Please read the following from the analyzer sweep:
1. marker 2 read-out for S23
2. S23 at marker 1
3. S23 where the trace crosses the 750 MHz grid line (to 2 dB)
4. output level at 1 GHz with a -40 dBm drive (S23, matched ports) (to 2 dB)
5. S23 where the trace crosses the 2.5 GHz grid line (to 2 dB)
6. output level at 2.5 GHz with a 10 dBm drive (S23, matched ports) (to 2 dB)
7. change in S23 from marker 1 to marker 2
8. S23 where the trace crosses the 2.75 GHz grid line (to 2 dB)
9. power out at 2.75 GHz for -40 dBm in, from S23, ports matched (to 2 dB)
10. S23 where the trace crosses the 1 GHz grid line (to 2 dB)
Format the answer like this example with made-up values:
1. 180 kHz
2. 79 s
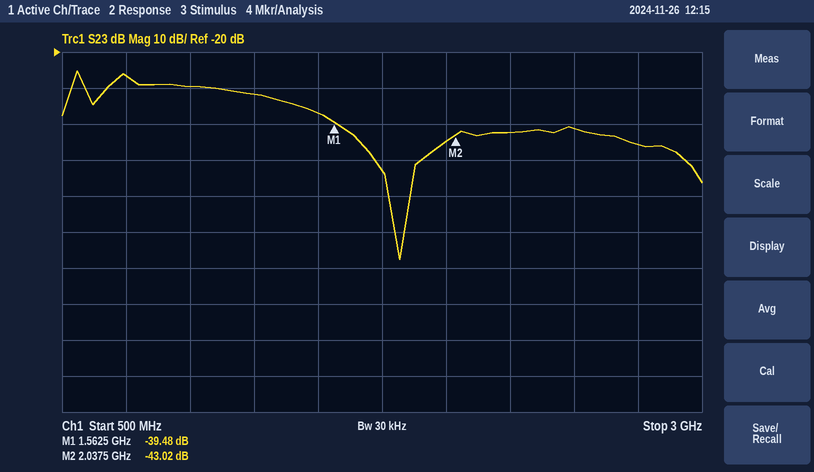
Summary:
1. -43.02 dB
2. -39.48 dB
3. -26 dB
4. -70 dBm
5. -42 dB
6. -32 dBm
7. -3.54 dB
8. -46 dB
9. -86 dBm
10. -30 dB
